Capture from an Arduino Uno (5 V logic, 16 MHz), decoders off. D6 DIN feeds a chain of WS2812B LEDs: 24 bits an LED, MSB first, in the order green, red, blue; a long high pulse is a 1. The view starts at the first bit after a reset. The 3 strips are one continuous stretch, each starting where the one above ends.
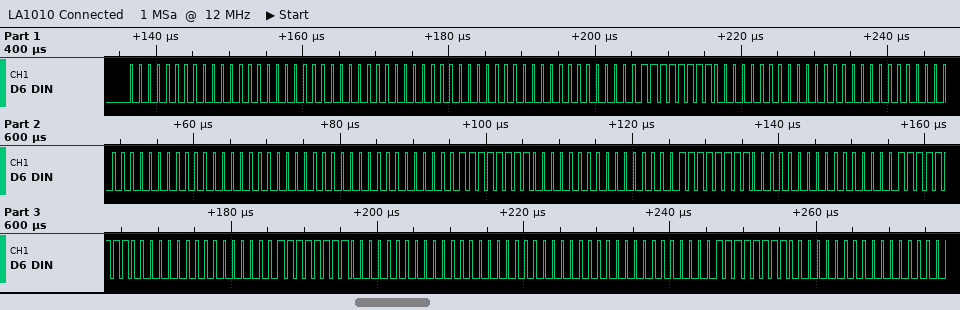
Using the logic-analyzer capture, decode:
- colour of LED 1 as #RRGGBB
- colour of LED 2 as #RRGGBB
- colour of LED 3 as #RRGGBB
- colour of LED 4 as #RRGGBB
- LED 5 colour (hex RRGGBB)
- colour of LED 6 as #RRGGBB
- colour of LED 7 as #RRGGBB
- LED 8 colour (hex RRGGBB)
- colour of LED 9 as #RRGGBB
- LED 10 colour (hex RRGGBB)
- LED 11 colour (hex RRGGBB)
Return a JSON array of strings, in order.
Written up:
["#000000", "#000000", "#FF0000", "#000000", "#000000", "#FF0000", "#FF0000", "#FF0000", "#FF0000", "#000000", "#FF0000"]
